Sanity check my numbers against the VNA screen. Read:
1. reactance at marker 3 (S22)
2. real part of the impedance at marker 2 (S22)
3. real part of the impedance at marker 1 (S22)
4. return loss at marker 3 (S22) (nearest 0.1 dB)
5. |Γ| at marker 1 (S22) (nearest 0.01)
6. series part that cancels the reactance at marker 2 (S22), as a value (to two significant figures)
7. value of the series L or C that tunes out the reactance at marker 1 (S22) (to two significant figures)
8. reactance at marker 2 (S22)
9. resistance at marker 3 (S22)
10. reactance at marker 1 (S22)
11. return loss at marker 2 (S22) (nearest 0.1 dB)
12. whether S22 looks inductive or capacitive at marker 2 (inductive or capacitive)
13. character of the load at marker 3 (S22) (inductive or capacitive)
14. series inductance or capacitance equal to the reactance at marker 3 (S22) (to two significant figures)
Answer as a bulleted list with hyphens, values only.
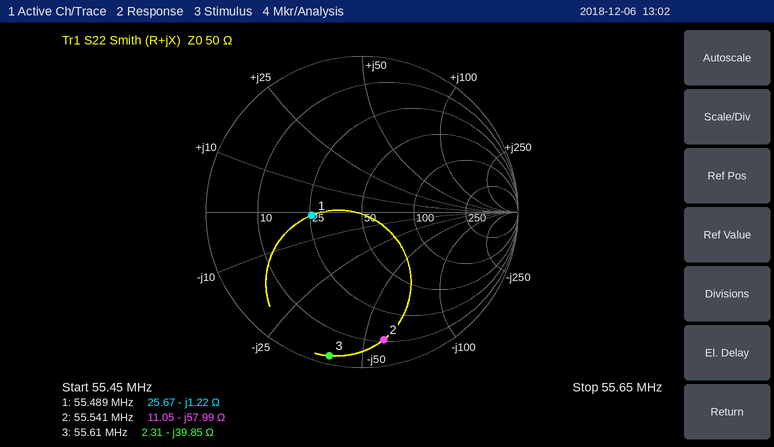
- -39.85 Ω
- 11.05 Ω
- 25.67 Ω
- 0.5 dB
- 0.32
- 170 nH
- 3.5 nH
- -57.99 Ω
- 2.31 Ω
- -1.22 Ω
- 1.6 dB
- capacitive
- capacitive
- 72 pF
